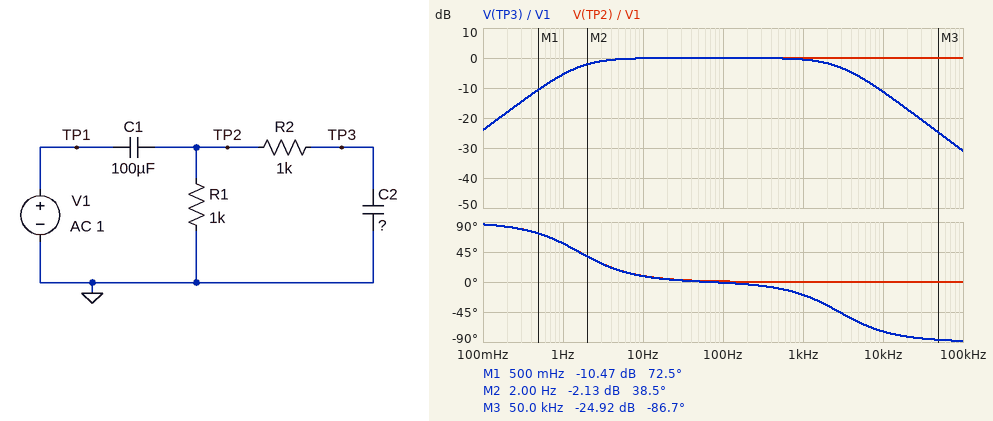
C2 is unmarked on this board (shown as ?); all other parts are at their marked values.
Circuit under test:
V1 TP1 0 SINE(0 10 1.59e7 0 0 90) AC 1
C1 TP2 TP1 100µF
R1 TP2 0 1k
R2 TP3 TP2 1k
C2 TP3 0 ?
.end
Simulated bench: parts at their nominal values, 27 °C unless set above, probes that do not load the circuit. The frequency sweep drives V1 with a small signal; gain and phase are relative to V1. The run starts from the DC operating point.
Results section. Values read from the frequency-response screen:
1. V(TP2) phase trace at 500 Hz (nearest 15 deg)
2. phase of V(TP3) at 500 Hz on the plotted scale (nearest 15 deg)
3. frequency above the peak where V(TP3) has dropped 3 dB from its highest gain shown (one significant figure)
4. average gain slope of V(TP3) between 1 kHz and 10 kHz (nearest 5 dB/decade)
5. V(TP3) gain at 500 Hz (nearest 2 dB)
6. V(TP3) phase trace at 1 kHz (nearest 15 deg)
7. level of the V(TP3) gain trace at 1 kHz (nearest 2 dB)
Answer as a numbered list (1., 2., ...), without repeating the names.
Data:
1. 0 deg
2. -15 deg
3. 3 kHz
4. -10 dB/decade
5. 0 dB
6. -15 deg
7. 0 dB
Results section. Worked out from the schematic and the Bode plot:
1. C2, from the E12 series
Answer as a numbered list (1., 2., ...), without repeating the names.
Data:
1. 56 nF
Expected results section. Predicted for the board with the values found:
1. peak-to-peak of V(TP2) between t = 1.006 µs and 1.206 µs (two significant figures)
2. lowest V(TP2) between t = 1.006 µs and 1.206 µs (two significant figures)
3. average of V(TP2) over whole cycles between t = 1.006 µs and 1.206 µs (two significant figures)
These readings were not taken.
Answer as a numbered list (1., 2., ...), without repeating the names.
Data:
1. 20 V
2. -20 V
3. -10 V
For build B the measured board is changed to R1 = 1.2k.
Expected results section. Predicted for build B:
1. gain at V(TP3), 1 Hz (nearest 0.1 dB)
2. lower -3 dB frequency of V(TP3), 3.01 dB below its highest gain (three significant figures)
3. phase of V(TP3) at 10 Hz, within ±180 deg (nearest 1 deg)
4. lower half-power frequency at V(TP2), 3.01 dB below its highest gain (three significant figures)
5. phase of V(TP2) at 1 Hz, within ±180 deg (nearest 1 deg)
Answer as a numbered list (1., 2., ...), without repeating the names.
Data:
1. -4.4 dB
2. 1.32 Hz
3. 7 deg
4. 1.33 Hz
5. 53 deg
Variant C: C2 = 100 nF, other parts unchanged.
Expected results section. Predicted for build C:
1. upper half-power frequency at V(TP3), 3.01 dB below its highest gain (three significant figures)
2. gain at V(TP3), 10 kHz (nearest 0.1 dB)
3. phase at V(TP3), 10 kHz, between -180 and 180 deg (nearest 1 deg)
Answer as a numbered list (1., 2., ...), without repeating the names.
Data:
1. 1.60 kHz
2. -16.1 dB
3. -81 deg
